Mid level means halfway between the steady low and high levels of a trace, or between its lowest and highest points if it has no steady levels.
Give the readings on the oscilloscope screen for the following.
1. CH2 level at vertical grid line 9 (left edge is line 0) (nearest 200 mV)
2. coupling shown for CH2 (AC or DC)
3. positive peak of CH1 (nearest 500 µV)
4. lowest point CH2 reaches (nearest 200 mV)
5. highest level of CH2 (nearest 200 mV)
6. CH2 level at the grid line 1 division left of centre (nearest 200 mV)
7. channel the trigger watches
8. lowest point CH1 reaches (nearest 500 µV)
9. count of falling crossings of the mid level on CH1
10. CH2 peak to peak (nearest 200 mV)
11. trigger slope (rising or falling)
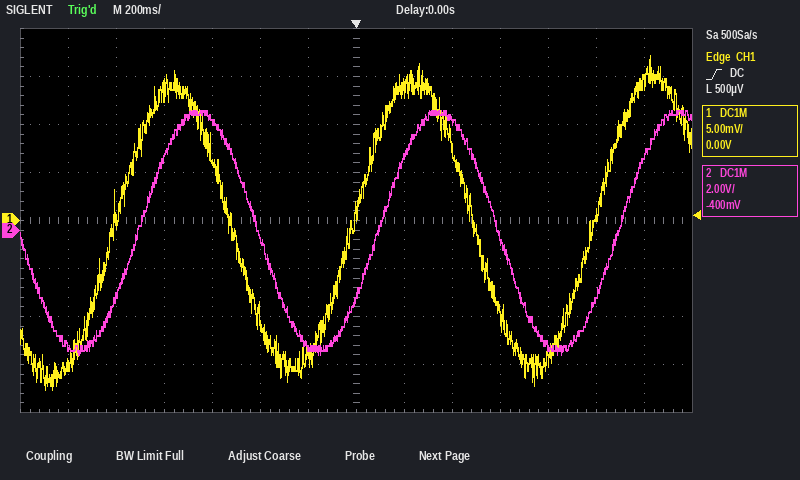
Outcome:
4.6 V
DC
17.0 mV
-5.2 V
5.0 V
-4.8 V
CH1
-17.5 mV
2
10.2 V
rising
